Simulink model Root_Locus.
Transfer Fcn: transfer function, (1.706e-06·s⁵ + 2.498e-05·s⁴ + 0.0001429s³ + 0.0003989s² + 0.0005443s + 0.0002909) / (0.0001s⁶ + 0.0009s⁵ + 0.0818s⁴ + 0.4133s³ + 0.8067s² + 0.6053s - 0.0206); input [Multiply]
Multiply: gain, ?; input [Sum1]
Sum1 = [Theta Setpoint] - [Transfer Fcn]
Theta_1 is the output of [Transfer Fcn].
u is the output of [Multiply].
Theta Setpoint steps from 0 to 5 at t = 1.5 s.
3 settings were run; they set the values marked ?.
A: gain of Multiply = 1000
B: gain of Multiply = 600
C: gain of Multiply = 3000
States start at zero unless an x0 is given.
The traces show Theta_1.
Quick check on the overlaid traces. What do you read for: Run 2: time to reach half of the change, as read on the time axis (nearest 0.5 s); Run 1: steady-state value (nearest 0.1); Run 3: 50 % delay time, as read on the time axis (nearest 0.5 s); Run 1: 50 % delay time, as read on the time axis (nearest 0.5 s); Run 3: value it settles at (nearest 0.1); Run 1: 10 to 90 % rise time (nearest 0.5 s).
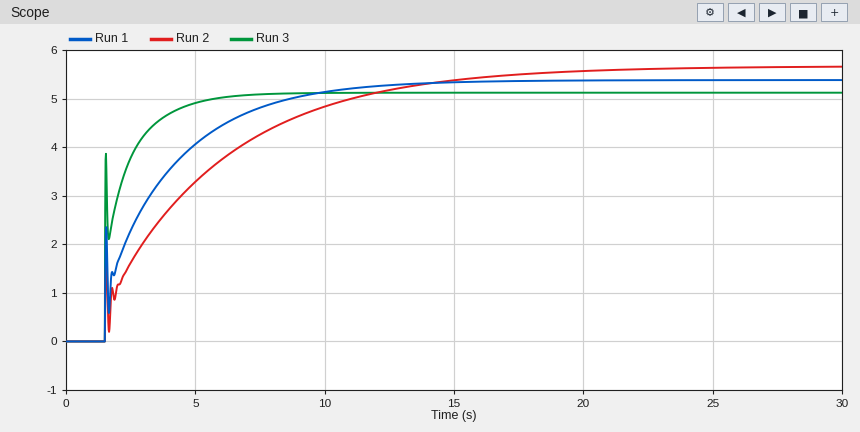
4.0 s
5.4
1.5 s
3.0 s
5.1
6.0 s
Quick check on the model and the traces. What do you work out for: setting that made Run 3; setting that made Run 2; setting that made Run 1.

C
B
A
